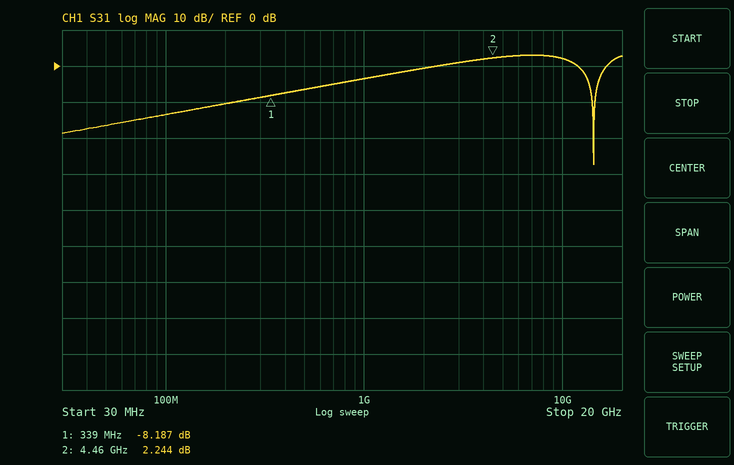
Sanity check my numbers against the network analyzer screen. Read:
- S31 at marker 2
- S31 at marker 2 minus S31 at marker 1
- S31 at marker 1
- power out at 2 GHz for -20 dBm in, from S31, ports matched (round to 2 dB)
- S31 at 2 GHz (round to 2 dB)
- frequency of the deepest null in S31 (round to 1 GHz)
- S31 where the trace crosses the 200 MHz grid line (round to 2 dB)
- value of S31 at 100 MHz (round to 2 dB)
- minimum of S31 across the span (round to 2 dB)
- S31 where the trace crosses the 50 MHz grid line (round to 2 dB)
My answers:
2.244 dB
10.431 dB
-8.187 dB
-20 dBm
0 dB
14 GHz
-10 dB
-14 dB
-28 dB
-16 dB
